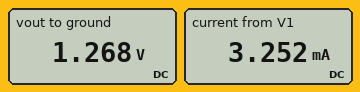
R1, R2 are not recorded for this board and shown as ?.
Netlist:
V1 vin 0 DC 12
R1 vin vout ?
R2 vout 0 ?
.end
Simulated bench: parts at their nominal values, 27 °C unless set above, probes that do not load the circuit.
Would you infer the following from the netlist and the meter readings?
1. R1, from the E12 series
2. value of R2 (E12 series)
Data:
3.3 kΩ
390 Ω
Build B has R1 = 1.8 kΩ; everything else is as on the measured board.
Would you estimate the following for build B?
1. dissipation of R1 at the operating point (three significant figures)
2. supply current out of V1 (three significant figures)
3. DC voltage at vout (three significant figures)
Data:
54.0 mW
5.48 mA
2.14 V
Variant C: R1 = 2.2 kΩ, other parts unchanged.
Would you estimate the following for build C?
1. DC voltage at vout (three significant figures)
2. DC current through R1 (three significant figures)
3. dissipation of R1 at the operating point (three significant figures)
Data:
1.81 V
4.63 mA
47.2 mW
